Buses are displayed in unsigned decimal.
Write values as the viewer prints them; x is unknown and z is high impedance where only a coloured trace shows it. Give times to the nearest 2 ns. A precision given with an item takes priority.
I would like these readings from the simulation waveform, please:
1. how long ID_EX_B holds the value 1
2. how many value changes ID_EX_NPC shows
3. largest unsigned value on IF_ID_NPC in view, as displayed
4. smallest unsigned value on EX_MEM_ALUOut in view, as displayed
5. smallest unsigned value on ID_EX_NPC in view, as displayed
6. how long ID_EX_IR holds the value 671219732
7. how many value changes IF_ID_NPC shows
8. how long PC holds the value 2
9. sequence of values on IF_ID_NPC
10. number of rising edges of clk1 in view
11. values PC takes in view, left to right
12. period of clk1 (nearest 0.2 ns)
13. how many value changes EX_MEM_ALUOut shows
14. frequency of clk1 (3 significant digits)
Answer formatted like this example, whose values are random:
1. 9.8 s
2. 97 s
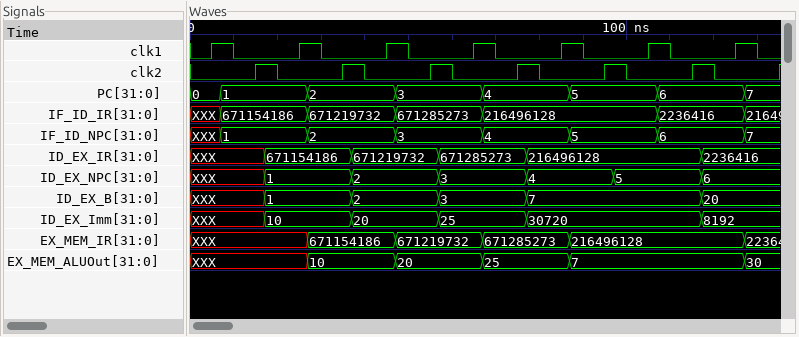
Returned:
1. 20 ns
2. 6
3. 7
4. 7
5. 1
6. 20 ns
7. 7
8. 20 ns
9. XXX, 1, 2, 3, 4, 5, 6, 7
10. 7
11. 0, 1, 2, 3, 4, 5, 6, 7
12. 20 ns
13. 5
14. 50.0 MHz
